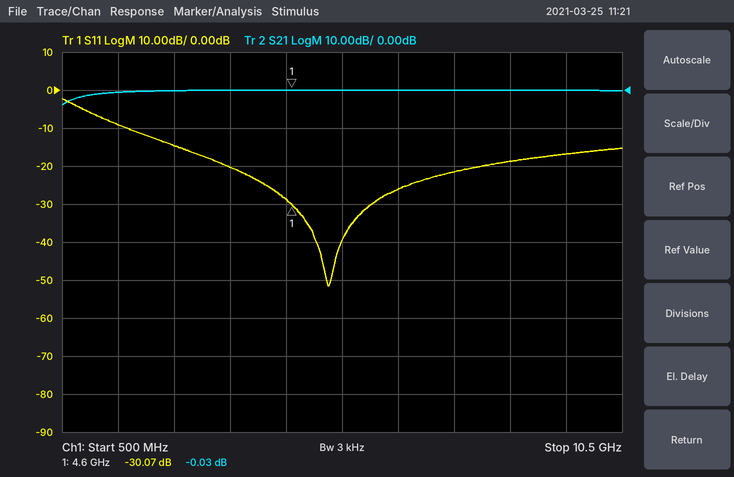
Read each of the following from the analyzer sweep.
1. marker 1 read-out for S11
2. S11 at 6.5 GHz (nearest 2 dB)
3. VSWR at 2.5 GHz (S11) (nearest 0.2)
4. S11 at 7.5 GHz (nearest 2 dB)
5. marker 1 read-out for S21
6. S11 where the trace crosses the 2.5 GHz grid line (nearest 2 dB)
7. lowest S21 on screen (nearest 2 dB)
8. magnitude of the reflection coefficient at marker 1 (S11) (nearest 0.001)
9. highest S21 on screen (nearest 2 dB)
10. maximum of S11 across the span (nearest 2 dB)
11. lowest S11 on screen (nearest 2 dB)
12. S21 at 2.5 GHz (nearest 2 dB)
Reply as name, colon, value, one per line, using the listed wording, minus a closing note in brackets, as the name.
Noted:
marker 1 read-out for S11: -30.07 dB
S11 at 6.5 GHz: -26 dB
VSWR at 2.5 GHz (S11): 1.4
S11 at 7.5 GHz: -22 dB
marker 1 read-out for S21: -0.03 dB
S11 where the trace crosses the 2.5 GHz grid line: -14 dB
lowest S21 on screen: -4 dB
magnitude of the reflection coefficient at marker 1 (S11): 0.031
highest S21 on screen: 0 dB
maximum of S11 across the span: -2 dB
lowest S11 on screen: -52 dB
S21 at 2.5 GHz: 0 dB
